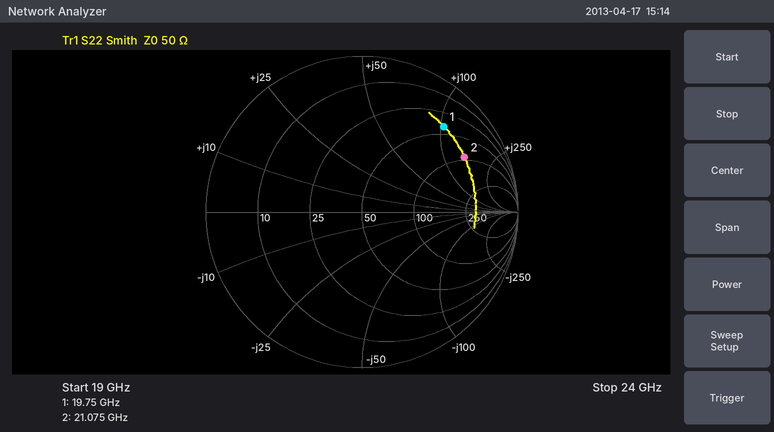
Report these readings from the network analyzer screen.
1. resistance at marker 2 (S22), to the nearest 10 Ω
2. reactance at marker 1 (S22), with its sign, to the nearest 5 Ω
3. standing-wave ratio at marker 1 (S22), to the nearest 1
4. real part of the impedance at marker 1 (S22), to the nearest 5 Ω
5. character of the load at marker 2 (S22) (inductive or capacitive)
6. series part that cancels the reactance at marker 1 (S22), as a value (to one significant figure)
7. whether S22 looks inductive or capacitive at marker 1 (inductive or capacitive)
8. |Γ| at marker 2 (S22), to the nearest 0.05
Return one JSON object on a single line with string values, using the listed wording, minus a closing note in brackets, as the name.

{"resistance at marker 2 (S22), to the nearest 10 Ω": "90 Ω", "reactance at marker 1 (S22), with its sign, to the nearest 5 Ω": "+105 Ω", "standing-wave ratio at marker 1 (S22), to the nearest 1": "7", "real part of the impedance at marker 1 (S22), to the nearest 5 Ω": "40 Ω", "character of the load at marker 2 (S22)": "inductive", "series part that cancels the reactance at marker 1 (S22), as a value": "80 fF", "whether S22 looks inductive or capacitive at marker 1": "inductive", "|Γ| at marker 2 (S22), to the nearest 0.05": "0.75"}
